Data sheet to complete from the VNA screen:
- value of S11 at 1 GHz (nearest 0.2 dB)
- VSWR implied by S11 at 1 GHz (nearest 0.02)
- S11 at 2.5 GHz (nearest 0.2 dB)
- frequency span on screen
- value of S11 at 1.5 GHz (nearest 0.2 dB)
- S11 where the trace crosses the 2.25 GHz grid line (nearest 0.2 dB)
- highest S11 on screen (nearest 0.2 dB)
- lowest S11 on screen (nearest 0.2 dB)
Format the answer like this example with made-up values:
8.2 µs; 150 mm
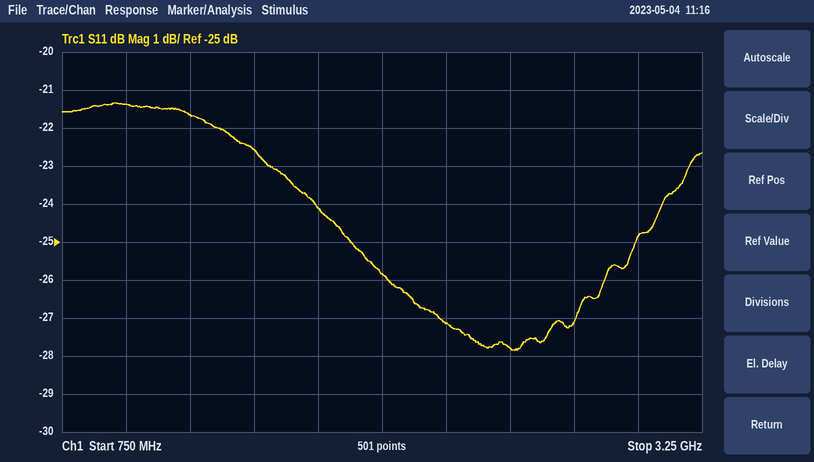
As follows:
-21.4 dB; 1.18; -27.8 dB; 2.5 GHz; -22.6 dB; -27.2 dB; -21.4 dB; -27.8 dB
